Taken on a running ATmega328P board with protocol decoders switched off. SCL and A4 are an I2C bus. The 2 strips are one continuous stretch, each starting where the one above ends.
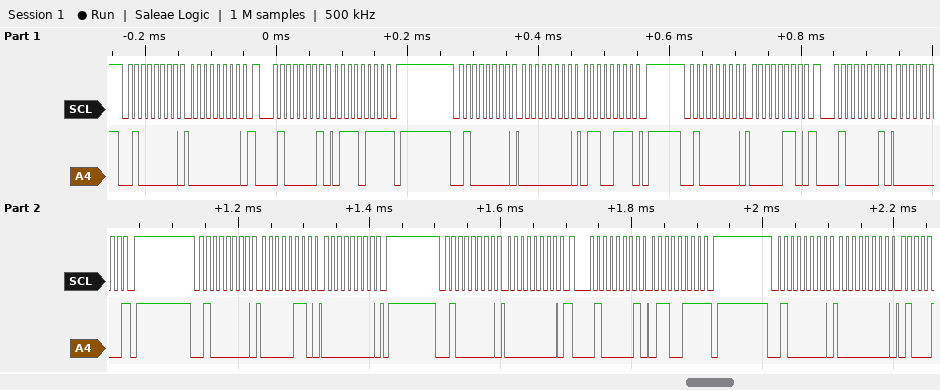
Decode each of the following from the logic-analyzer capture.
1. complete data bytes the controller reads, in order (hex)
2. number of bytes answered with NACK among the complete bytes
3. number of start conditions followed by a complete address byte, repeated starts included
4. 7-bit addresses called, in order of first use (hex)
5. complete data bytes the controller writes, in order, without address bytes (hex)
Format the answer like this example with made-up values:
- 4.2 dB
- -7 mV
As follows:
- 77 00 67
- 3
- 9
- 0x20
- 00 00 67 06 06 00 00 00
